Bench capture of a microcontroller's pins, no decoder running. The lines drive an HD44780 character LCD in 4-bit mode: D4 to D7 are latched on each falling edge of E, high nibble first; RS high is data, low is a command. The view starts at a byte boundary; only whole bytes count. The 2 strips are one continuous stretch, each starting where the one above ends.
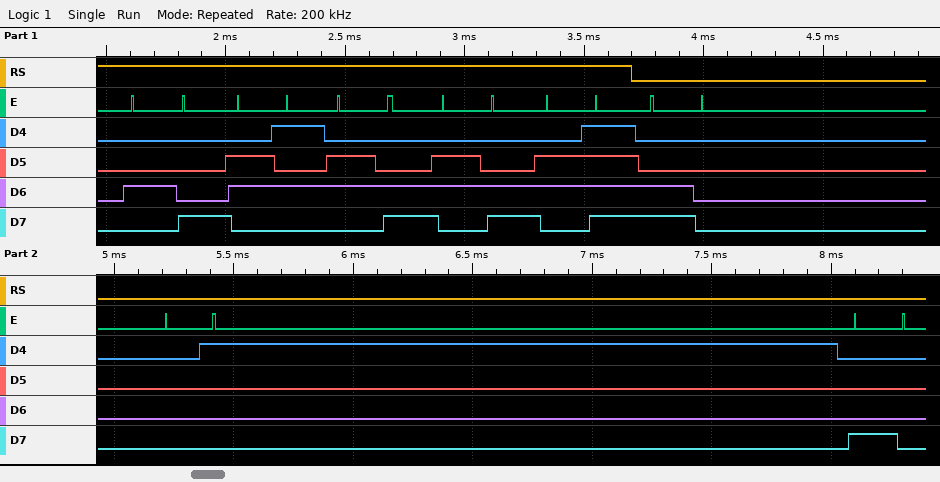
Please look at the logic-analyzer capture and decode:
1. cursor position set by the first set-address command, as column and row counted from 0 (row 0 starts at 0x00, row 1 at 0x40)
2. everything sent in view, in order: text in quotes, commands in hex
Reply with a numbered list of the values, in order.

1. column 0, row 1
2. "Hello" 0xC0 0x01 0x80
